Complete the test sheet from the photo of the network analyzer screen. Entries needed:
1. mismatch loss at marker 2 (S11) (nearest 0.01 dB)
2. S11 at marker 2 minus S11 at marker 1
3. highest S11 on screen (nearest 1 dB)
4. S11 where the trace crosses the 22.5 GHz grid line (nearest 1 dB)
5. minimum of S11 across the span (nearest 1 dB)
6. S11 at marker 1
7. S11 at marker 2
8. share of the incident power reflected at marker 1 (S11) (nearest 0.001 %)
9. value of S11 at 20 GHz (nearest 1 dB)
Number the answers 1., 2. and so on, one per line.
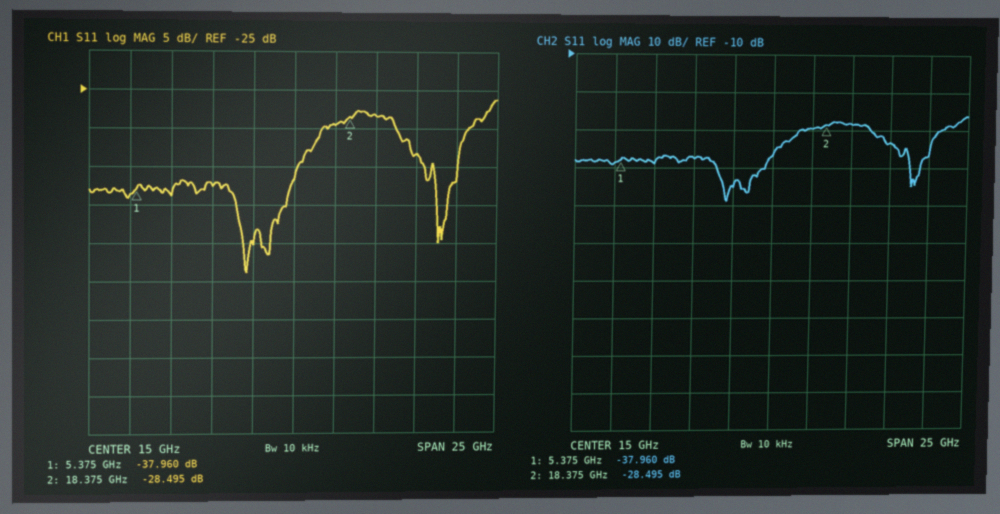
1. 0.01 dB
2. 9.465 dB
3. -26 dB
4. -33 dB
5. -49 dB
6. -37.960 dB
7. -28.495 dB
8. 0.016 %
9. -28 dB
